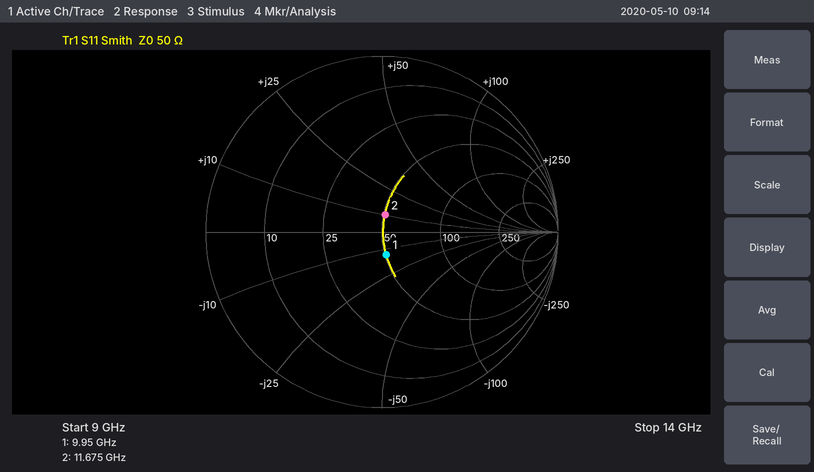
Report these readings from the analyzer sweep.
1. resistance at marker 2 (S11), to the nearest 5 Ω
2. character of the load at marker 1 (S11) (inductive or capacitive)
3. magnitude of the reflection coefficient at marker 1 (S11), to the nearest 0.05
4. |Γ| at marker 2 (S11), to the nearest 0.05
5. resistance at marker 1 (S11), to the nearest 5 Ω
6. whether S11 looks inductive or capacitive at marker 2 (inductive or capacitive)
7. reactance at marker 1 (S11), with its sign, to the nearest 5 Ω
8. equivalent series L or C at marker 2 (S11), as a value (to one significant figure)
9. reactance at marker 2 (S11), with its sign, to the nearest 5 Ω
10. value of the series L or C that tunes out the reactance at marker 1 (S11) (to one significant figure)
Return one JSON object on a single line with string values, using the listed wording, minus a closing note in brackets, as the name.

{"resistance at marker 2 (S11), to the nearest 5 Ω": "50 Ω", "character of the load at marker 1 (S11)": "capacitive", "magnitude of the reflection coefficient at marker 1 (S11), to the nearest 0.05": "0.15", "|Γ| at marker 2 (S11), to the nearest 0.05": "0.10", "resistance at marker 1 (S11), to the nearest 5 Ω": "50 Ω", "whether S11 looks inductive or capacitive at marker 2": "inductive", "reactance at marker 1 (S11), with its sign, to the nearest 5 Ω": "-15 Ω", "equivalent series L or C at marker 2 (S11), as a value": "100 pH", "reactance at marker 2 (S11), with its sign, to the nearest 5 Ω": "+10 Ω", "value of the series L or C that tunes out the reactance at marker 1 (S11)": "200 pH"}
